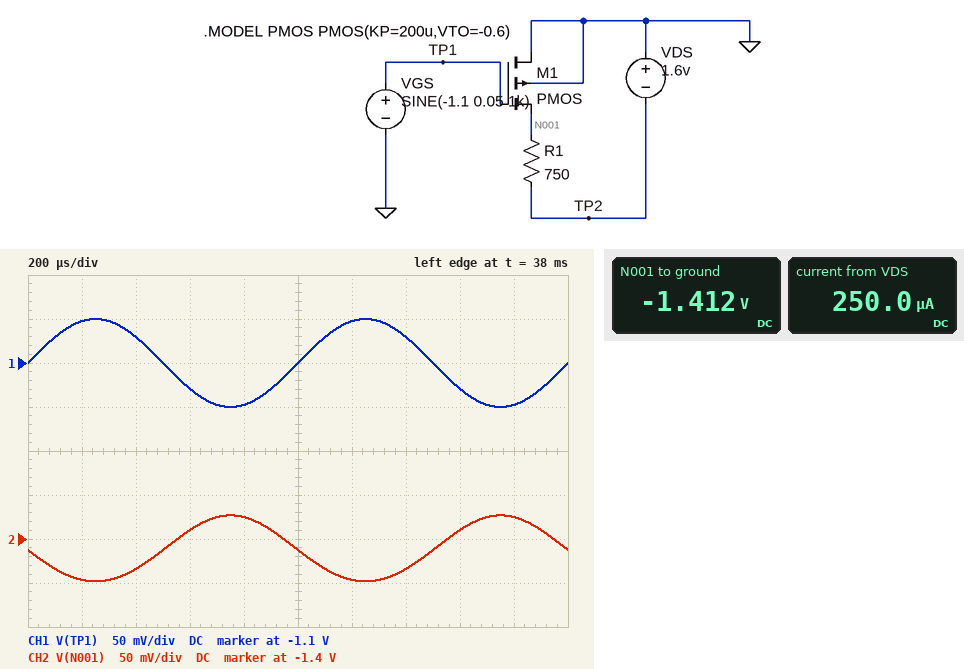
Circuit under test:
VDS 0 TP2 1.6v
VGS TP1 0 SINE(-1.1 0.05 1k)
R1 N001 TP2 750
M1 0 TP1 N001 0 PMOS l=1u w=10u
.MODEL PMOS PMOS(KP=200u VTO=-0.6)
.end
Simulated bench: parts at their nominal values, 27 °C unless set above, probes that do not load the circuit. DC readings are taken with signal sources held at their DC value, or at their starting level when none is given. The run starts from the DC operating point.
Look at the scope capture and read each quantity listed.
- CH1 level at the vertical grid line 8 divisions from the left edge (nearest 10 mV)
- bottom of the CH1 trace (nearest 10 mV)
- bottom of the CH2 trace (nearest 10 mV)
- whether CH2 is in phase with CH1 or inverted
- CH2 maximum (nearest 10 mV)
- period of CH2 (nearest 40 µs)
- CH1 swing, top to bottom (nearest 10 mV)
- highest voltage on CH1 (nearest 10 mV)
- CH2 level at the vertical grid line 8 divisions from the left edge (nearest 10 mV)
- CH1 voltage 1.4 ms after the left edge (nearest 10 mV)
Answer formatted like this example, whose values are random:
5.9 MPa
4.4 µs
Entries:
-1.13 V
-1.15 V
-1.45 V
inverted
-1.37 V
1.00 ms
100 mV
-1.05 V
-1.39 V
-1.07 V
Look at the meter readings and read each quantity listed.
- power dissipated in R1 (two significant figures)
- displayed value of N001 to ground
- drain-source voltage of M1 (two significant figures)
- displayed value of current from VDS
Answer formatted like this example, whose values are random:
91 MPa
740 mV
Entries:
47 µW
-1.412 V
1.4 V
250.0 µA
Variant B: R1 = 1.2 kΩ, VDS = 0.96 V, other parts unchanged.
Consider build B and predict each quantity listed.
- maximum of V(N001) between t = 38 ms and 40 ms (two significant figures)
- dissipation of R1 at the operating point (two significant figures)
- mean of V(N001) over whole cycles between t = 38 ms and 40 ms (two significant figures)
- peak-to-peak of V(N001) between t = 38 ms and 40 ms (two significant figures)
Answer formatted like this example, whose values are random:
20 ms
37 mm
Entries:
-600 mV
75 µW
-660 mV
120 mV
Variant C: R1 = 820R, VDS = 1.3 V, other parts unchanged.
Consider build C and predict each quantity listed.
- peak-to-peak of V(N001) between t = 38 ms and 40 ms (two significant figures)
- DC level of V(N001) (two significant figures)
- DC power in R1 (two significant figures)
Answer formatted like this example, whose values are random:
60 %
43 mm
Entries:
82 mV
-1.1 V
51 µW
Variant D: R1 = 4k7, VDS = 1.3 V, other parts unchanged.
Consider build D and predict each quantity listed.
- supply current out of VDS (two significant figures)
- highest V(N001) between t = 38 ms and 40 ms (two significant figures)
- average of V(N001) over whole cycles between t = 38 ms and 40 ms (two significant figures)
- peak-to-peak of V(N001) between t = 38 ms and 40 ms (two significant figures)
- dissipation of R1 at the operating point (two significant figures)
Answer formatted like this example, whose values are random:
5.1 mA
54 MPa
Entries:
210 µA
-260 mV
-310 mV
110 mV
210 µW
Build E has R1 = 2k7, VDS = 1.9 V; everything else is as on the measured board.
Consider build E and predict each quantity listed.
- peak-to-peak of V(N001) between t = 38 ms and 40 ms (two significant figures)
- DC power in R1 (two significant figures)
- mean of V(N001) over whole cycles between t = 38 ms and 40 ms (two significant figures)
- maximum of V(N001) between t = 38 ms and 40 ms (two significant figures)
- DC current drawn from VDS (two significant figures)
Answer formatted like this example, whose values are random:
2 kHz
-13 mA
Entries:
270 mV
170 µW
-1.2 V
-1.1 V
250 µA
